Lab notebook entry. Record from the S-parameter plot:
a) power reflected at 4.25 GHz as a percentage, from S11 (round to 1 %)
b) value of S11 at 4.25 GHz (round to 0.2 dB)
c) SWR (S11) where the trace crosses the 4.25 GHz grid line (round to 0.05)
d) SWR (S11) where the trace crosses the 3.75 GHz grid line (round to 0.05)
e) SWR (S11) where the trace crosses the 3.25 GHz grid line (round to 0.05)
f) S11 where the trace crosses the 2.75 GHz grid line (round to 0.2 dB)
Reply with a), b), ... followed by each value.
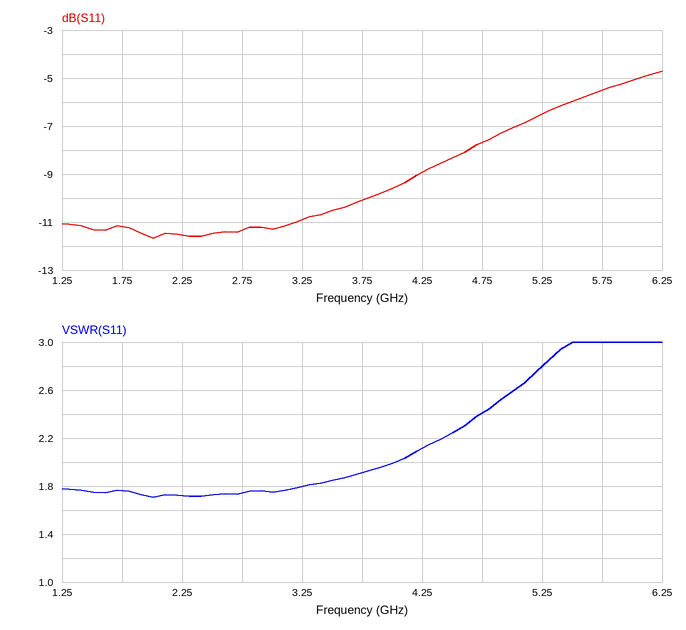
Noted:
a) 13 %
b) -9.0 dB
c) 2.10
d) 1.90
e) 1.80
f) -11.4 dB
